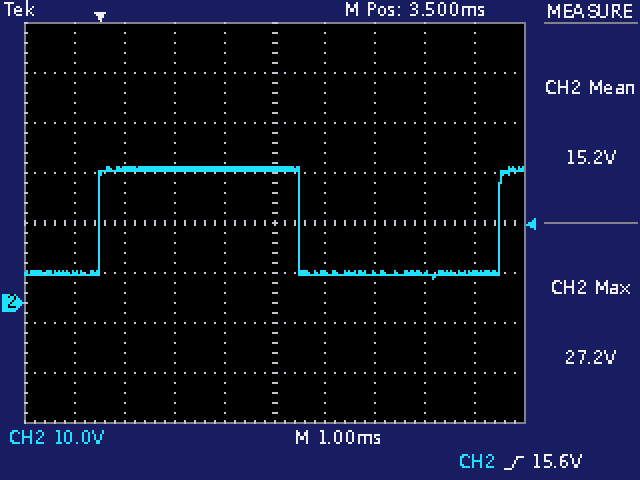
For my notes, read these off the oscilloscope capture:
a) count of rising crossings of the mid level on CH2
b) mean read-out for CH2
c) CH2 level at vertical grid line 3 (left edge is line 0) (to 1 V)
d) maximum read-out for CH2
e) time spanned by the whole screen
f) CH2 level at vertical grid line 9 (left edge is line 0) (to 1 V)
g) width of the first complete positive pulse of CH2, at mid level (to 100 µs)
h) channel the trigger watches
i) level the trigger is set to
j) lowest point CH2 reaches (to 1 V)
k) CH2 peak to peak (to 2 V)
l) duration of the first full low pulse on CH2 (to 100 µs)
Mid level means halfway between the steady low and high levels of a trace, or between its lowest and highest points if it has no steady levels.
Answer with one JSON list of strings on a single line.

["2", "15.2 V", "27 V", "27.2 V", "10 ms", "6 V", "4.0 ms", "CH2", "15.6 V", "5 V", "22 V", "4.0 ms"]
